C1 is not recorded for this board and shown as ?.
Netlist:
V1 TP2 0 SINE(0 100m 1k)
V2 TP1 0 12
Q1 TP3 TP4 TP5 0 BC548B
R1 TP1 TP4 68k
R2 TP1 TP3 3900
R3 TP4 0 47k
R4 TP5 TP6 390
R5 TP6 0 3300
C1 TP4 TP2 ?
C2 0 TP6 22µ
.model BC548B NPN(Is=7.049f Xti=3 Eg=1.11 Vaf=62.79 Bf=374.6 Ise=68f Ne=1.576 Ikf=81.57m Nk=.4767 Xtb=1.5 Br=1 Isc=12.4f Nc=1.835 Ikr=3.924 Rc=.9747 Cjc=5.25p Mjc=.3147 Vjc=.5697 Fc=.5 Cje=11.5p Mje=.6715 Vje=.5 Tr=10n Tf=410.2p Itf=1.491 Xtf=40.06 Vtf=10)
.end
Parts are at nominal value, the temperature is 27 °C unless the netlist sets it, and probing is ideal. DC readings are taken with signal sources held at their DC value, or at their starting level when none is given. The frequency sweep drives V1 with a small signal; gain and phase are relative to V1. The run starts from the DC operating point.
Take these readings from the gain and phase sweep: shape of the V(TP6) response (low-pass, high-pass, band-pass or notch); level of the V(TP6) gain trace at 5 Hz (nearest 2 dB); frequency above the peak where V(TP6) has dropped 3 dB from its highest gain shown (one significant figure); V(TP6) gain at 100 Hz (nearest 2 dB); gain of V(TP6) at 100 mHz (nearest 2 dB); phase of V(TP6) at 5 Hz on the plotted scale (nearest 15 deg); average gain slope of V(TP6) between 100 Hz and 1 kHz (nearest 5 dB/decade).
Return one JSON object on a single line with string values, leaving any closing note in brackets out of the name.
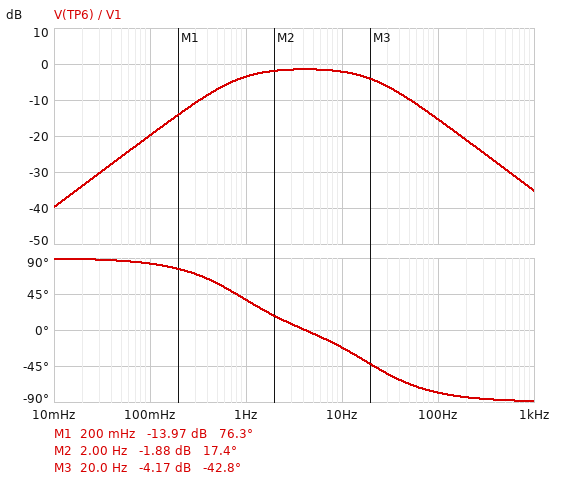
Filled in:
{"shape of the V(TP6) response": "band-pass", "level of the V(TP6) gain trace at 5 Hz": "-2 dB", "frequency above the peak where V(TP6) has dropped 3 dB from its highest gain shown": "20 Hz", "V(TP6) gain at 100 Hz": "-16 dB", "gain of V(TP6) at 100 mHz": "-20 dB", "phase of V(TP6) at 5 Hz on the plotted scale": "0 deg", "average gain slope of V(TP6) between 100 Hz and 1 kHz": "-20 dB/decade"}
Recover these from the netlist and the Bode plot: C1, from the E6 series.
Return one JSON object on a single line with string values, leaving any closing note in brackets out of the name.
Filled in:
{"C1, from the E6 series": "6.8 µF"}
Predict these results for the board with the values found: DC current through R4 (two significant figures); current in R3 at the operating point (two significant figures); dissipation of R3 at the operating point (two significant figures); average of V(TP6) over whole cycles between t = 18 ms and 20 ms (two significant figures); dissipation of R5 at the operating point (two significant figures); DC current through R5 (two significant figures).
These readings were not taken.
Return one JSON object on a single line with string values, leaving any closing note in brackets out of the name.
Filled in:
{"DC current through R4": "1.1 mA", "current in R3 at the operating point": "100 µA", "dissipation of R3 at the operating point": "490 µW", "average of V(TP6) over whole cycles between t = 18 ms and 20 ms": "3.7 V", "dissipation of R5 at the operating point": "4.1 mW", "DC current through R5": "1.1 mA"}
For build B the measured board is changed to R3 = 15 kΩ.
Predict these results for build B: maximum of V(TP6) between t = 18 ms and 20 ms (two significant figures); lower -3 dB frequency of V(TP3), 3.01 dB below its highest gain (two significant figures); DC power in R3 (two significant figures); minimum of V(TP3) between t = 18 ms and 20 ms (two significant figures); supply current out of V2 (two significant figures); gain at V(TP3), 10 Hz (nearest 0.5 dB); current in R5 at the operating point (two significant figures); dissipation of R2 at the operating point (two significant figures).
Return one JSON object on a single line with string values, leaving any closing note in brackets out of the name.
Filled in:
{"maximum of V(TP6) between t = 18 ms and 20 ms": "1.4 V", "lower -3 dB frequency of V(TP3), 3.01 dB below its highest gain": "18 Hz", "DC power in R3": "310 µW", "minimum of V(TP3) between t = 18 ms and 20 ms": "9.5 V", "supply current out of V2": "550 µA", "gain at V(TP3), 10 Hz": "12.5 dB", "current in R5 at the operating point": "410 µA", "dissipation of R2 at the operating point": "650 µW"}
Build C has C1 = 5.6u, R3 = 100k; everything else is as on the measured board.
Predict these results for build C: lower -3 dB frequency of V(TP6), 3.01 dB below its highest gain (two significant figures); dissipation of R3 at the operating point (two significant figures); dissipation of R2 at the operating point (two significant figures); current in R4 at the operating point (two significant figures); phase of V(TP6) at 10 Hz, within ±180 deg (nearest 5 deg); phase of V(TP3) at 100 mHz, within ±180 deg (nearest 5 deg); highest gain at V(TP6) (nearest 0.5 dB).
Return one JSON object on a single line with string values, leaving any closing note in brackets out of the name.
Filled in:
{"lower -3 dB frequency of V(TP6), 3.01 dB below its highest gain": "2.8 Hz", "dissipation of R3 at the operating point": "420 µW", "dissipation of R2 at the operating point": "9.4 mW", "current in R4 at the operating point": "1.6 mA", "phase of V(TP6) at 10 Hz, within ±180 deg": "10 deg", "phase of V(TP3) at 100 mHz, within ±180 deg": "85 deg", "highest gain at V(TP6)": "-12.0 dB"}
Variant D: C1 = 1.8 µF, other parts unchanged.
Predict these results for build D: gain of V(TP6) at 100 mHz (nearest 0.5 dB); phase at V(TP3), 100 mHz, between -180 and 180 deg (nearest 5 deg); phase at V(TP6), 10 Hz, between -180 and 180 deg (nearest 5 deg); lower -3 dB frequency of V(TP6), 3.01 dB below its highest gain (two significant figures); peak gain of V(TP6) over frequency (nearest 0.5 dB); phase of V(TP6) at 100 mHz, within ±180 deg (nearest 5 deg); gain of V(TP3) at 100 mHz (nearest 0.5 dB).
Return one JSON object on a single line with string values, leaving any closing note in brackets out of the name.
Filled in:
{"gain of V(TP6) at 100 mHz": "-31.5 dB", "phase at V(TP3), 100 mHz, between -180 and 180 deg": "-90 deg", "phase at V(TP6), 10 Hz, between -180 and 180 deg": "-10 deg", "lower -3 dB frequency of V(TP6), 3.01 dB below its highest gain": "2.5 Hz", "peak gain of V(TP6) over frequency": "-2.5 dB", "phase of V(TP6) at 100 mHz, within ±180 deg": "90 deg", "gain of V(TP3) at 100 mHz": "-30.0 dB"}
